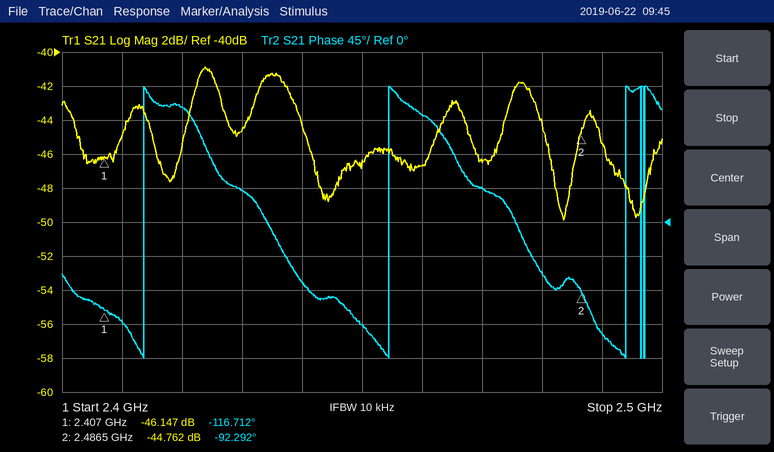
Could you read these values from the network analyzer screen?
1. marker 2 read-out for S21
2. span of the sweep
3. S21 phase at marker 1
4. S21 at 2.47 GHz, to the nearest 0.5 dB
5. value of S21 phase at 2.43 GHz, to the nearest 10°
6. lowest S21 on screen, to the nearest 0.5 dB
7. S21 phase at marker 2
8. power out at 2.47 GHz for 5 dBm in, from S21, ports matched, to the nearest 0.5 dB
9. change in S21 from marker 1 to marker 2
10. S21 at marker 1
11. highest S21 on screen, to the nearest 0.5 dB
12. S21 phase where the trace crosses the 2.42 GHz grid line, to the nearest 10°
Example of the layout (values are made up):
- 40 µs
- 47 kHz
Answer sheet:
- -44.762 dB
- 100 MHz
- -116.712°
- -46.5 dB
- 40°
- -50.0 dB
- -92.292°
- -41.5 dBm
- 1.385 dB
- -46.147 dB
- -41.0 dB
- 150°
